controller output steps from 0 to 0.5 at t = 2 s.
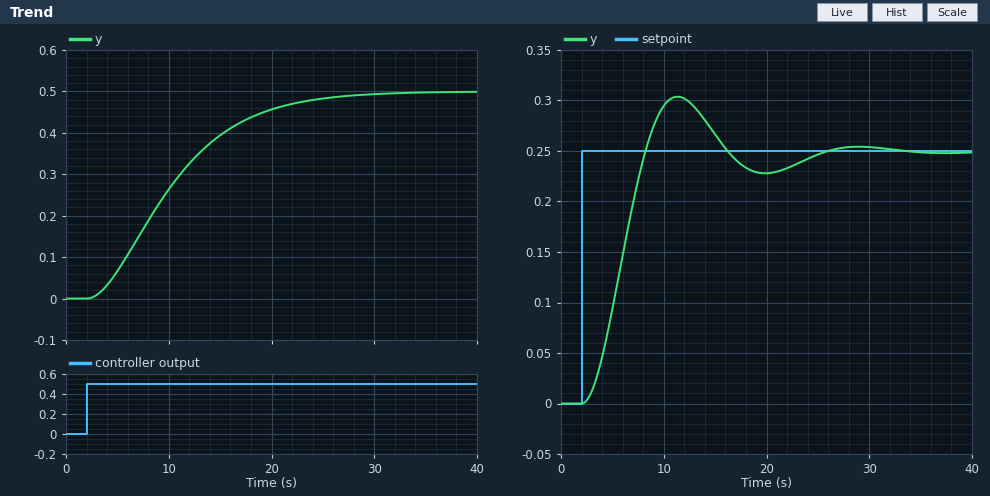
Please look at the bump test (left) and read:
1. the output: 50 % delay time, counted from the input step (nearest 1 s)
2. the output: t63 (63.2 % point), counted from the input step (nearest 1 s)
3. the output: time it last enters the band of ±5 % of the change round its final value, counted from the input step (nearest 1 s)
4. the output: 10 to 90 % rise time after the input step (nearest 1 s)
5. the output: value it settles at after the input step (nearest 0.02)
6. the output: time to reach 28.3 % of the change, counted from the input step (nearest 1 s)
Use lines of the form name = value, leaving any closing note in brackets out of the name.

the output: 50 % delay time, counted from the input step = 8 s
the output: t63 (63.2 % point), counted from the input step = 10 s
the output: time it last enters the band of ±5 % of the change round its final value, counted from the input step = 21 s
the output: 10 to 90 % rise time after the input step = 15 s
the output: value it settles at after the input step = 0.50
the output: time to reach 28.3 % of the change, counted from the input step = 5 s
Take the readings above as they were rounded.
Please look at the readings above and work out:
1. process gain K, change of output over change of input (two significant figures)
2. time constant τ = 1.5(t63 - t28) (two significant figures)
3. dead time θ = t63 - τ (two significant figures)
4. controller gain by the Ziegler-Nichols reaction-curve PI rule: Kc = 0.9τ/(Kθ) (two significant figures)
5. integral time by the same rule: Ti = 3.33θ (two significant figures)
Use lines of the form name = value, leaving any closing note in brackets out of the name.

process gain K, change of output over change of input = 1.0
time constant τ = 1.5(t63 - t28) = 7.5 s
dead time θ = t63 - τ = 2.5 s
controller gain by the Ziegler-Nichols reaction-curve PI rule: Kc = 0.9τ/(Kθ) = 2.7
integral time by the same rule: Ti = 3.33θ = 8.3 s
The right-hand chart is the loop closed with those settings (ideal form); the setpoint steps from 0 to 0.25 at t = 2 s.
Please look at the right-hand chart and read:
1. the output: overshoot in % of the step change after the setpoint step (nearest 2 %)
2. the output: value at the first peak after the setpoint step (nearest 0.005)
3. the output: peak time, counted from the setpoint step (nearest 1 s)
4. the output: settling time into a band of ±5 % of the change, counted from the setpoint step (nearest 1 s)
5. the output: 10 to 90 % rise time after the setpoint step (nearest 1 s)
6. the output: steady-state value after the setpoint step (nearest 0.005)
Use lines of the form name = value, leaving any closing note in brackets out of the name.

the output: overshoot in % of the step change after the setpoint step = 22 %
the output: value at the first peak after the setpoint step = 0.305
the output: peak time, counted from the setpoint step = 9 s
the output: settling time into a band of ±5 % of the change, counted from the setpoint step = 21 s
the output: 10 to 90 % rise time after the setpoint step = 4 s
the output: steady-state value after the setpoint step = 0.250
